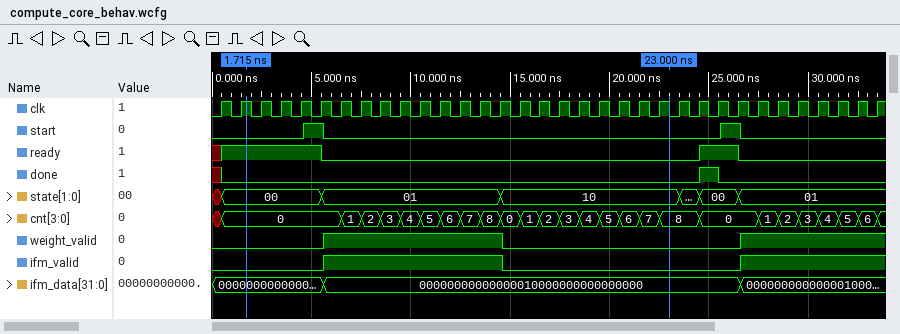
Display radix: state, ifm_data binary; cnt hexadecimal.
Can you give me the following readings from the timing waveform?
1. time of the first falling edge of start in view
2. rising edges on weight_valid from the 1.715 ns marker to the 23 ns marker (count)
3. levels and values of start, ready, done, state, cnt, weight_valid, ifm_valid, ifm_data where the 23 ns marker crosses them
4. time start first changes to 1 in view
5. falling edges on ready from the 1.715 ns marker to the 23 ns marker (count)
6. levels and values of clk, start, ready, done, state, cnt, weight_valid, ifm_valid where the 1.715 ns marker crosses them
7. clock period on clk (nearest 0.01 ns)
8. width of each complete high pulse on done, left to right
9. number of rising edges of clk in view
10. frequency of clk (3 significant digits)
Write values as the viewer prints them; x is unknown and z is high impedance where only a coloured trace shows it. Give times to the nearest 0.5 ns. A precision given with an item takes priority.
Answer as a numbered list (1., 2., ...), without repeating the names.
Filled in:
1. 5.5 ns
2. 1
3. start=0, ready=0, done=0, state=10, cnt=8, weight_valid=0, ifm_valid=0, ifm_data=00000000000000010000000000000000
4. 4.5 ns
5. 1
6. clk=1, start=0, ready=1, done=0, state=00, cnt=0, weight_valid=0, ifm_valid=0
7. 1 ns
8. 1 ns
9. 34
10. 1.00 GHz
